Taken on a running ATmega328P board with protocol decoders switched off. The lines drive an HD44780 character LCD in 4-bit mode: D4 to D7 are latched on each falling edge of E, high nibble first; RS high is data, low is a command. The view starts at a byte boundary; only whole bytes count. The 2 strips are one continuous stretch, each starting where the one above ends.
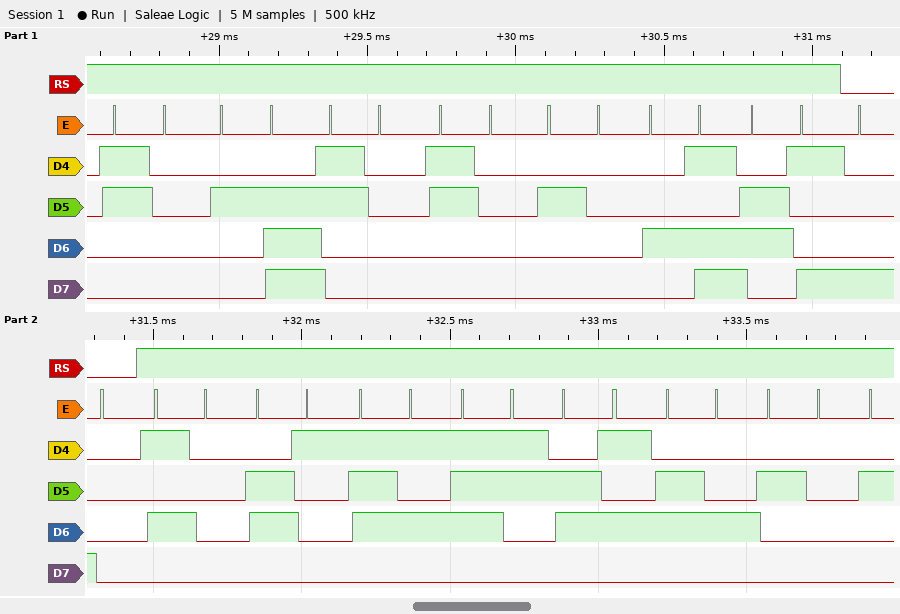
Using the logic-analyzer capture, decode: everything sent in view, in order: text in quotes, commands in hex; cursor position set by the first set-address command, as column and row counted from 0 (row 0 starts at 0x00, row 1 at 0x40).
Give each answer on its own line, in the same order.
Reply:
"0.00 Mi" 0x80 "Paused "
column 0, row 0
